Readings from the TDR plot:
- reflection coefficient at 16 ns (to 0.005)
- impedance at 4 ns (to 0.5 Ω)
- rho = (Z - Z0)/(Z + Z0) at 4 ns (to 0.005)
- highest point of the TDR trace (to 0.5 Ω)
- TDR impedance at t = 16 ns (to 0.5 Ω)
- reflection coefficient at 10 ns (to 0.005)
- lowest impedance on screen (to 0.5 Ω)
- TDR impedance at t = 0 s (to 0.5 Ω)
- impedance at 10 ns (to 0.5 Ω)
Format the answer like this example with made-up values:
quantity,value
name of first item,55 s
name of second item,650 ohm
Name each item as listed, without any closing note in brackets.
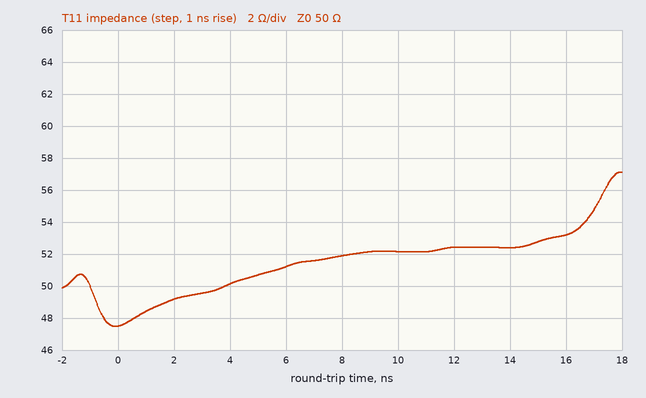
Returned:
quantity,value
reflection coefficient at 16 ns,+0.030
impedance at 4 ns,50.0 Ω
rho = (Z - Z0)/(Z + Z0) at 4 ns,0.000
highest point of the TDR trace,57.0 Ω
TDR impedance at t = 16 ns,53.0 Ω
reflection coefficient at 10 ns,+0.020
lowest impedance on screen,47.5 Ω
TDR impedance at t = 0 s,47.5 Ω
impedance at 10 ns,52.0 Ω
